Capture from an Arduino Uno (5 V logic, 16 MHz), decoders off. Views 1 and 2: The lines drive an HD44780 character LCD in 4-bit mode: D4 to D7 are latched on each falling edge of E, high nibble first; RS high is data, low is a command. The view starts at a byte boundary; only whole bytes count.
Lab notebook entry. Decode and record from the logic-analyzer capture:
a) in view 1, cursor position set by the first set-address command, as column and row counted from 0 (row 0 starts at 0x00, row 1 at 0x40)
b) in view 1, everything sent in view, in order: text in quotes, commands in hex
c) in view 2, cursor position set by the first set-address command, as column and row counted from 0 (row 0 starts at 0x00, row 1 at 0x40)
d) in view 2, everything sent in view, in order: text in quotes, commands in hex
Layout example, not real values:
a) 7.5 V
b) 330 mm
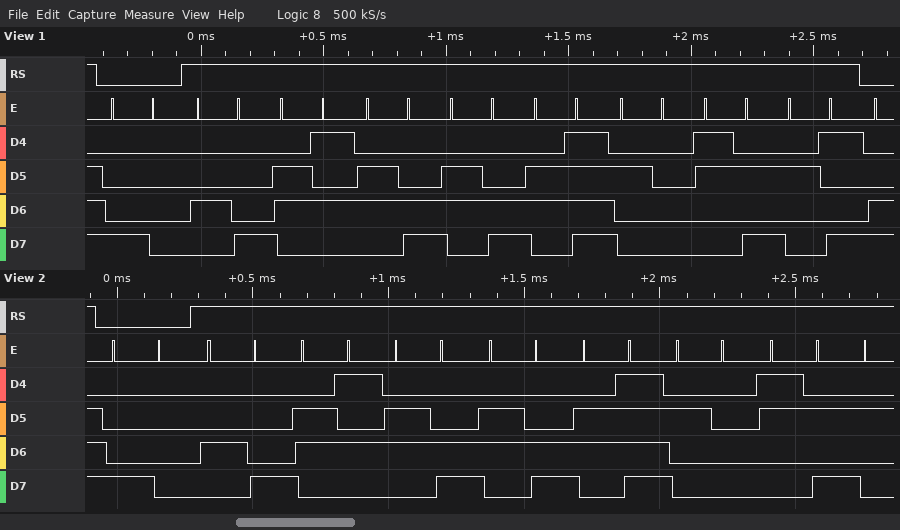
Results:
a) column 0, row 0
b) 0x80 "Hello :)"
c) column 0, row 0
d) 0x80 "Hello :"
